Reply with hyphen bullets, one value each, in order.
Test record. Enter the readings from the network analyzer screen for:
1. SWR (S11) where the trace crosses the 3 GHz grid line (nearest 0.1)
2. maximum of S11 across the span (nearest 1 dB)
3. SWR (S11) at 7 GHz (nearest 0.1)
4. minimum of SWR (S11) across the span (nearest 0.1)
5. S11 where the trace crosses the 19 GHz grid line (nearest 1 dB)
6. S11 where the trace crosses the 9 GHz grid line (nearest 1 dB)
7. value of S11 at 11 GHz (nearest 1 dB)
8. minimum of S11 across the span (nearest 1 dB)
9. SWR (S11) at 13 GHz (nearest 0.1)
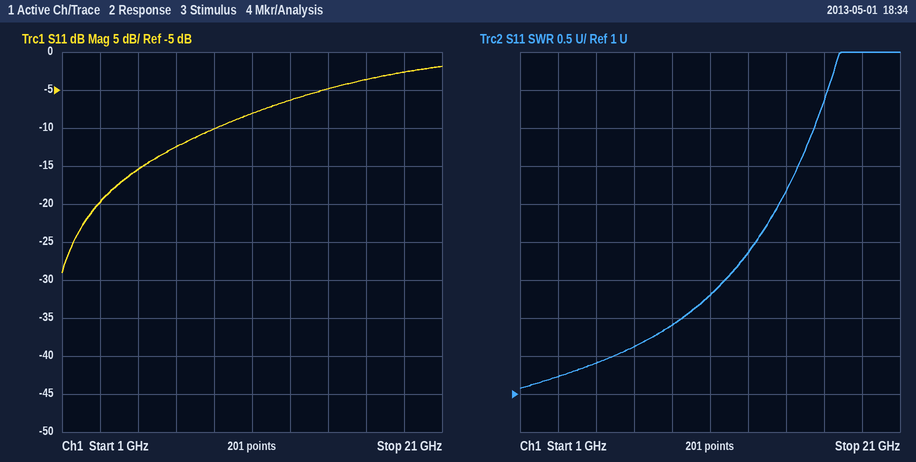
- 1.2
- -2 dB
- 1.6
- 1.1
- -3 dB
- -10 dB
- -8 dB
- -29 dB
- 2.9
